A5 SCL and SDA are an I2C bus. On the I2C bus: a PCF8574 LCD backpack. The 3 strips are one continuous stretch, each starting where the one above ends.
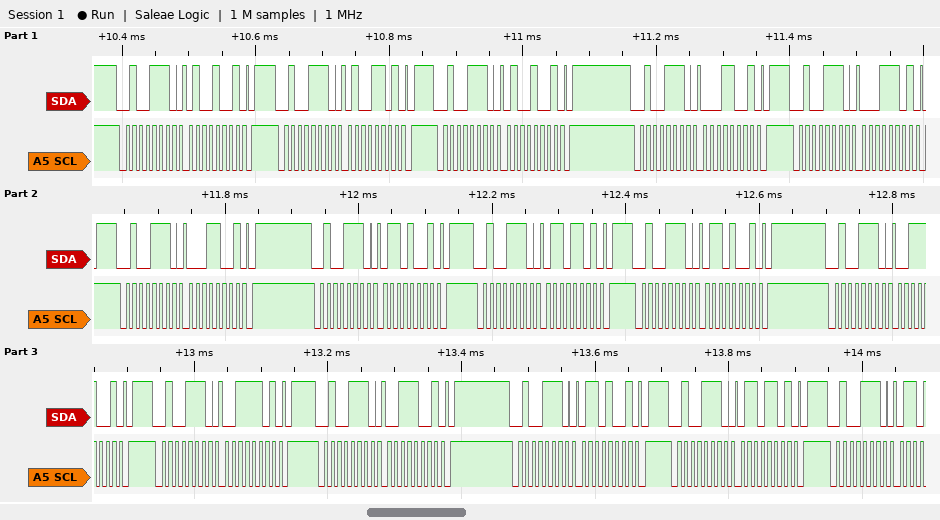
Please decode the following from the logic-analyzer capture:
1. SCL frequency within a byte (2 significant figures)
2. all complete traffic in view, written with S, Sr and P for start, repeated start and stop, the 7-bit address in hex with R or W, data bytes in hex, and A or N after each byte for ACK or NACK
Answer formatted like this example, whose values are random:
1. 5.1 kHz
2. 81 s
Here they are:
1. 100 kHz
2. S 27W A 49 A P S 27W A 4D A P S 27W A 49 A P S 27W A 19 A P S 27W A 1D A P S 27W A 19 A P S 27W A 69 A P S 27W A 6D A P S 27W A 69 A P S 27W A 39 A P S 27W A 3D A P S 27W A 39 A P S 27W A 69 A P S 27W A 6D A P S 27W A
